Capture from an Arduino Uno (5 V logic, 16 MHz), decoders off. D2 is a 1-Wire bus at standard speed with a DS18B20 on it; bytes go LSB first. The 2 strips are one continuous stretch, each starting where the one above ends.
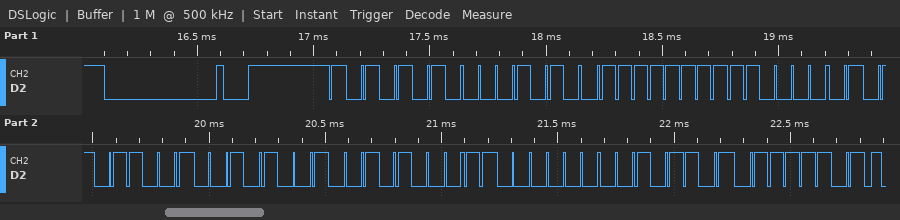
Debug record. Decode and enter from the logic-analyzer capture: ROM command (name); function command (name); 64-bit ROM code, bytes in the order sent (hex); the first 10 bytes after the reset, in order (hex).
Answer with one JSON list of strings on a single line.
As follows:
["Match ROM", "Read Scratchpad", "28 FF 83 9A 94 14 03 B4", "55 28 FF 83 9A 94 14 03 B4 BE"]
